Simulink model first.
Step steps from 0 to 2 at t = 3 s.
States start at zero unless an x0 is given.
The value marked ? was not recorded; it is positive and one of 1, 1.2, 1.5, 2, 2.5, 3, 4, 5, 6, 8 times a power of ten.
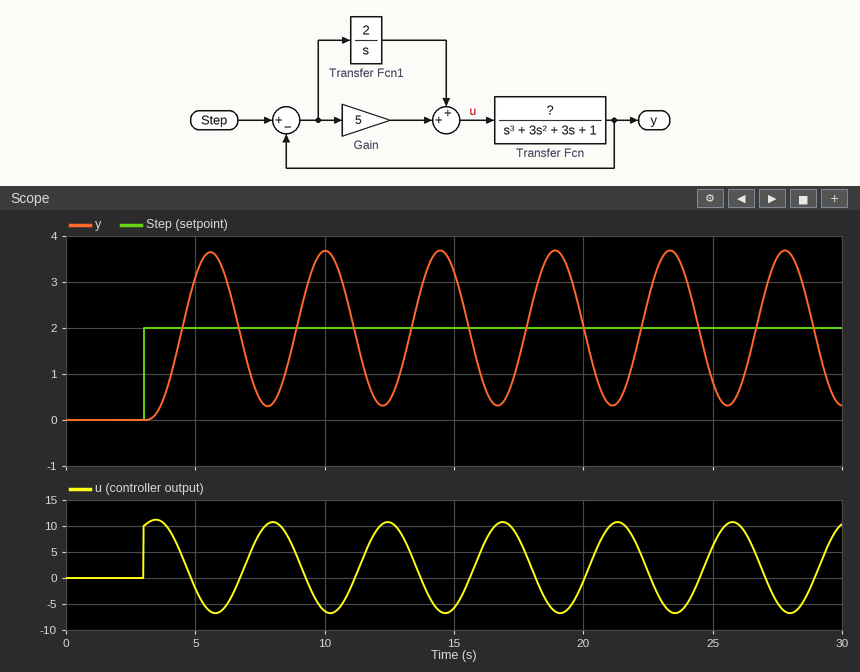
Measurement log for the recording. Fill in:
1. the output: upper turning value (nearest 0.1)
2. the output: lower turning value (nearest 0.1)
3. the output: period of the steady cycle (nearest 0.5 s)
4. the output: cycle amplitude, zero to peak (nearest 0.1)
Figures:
3.7
0.3
4.5 s
1.7
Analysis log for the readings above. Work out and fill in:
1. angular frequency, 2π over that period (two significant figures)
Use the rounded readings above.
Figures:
1.4 rad/s
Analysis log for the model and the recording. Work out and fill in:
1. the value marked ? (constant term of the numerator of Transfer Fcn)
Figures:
1
